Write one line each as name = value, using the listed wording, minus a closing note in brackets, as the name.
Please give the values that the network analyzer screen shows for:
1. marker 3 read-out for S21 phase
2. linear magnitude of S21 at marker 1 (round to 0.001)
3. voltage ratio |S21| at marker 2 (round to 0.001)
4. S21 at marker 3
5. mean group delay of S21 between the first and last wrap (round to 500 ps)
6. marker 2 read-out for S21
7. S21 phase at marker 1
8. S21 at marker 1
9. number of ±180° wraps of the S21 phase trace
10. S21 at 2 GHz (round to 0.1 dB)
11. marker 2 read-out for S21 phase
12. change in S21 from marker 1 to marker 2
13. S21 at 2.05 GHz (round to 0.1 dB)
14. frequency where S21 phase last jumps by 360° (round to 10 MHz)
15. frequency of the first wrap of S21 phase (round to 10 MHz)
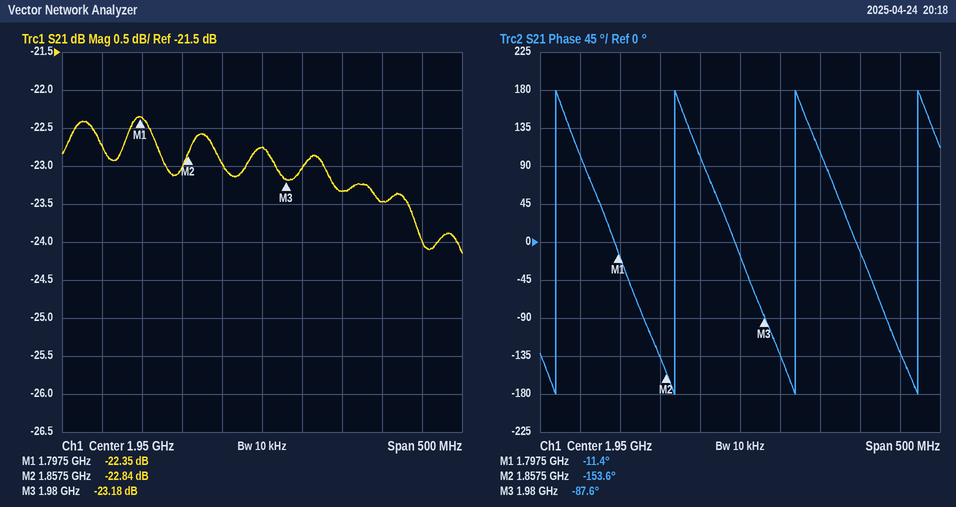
marker 3 read-out for S21 phase = -87.6°
linear magnitude of S21 at marker 1 = 0.076
voltage ratio |S21| at marker 2 = 0.072
S21 at marker 3 = -23.18 dB
mean group delay of S21 between the first and last wrap = 6.5 ns
marker 2 read-out for S21 = -22.84 dB
S21 phase at marker 1 = -11.4°
S21 at marker 1 = -22.35 dB
number of ±180° wraps of the S21 phase trace = 4
S21 at 2 GHz = -23.0 dB
marker 2 read-out for S21 phase = -153.6°
change in S21 from marker 1 to marker 2 = -0.49 dB
S21 at 2.05 GHz = -23.3 dB
frequency where S21 phase last jumps by 360° = 2.17 GHz
frequency of the first wrap of S21 phase = 1.72 GHz
